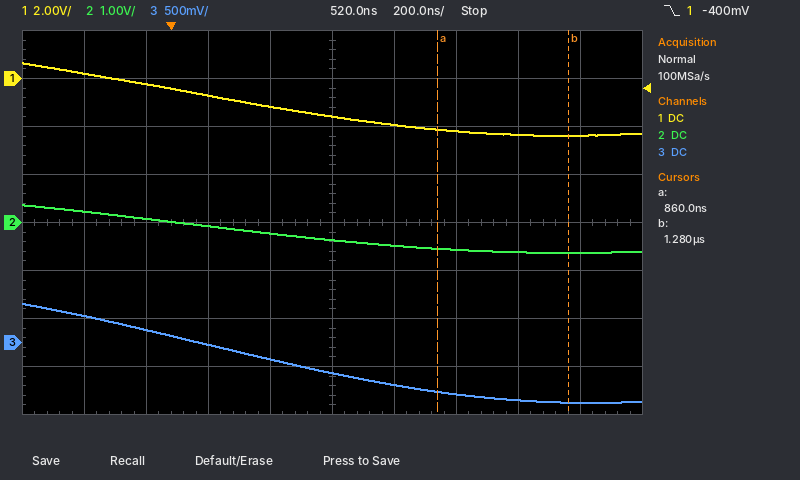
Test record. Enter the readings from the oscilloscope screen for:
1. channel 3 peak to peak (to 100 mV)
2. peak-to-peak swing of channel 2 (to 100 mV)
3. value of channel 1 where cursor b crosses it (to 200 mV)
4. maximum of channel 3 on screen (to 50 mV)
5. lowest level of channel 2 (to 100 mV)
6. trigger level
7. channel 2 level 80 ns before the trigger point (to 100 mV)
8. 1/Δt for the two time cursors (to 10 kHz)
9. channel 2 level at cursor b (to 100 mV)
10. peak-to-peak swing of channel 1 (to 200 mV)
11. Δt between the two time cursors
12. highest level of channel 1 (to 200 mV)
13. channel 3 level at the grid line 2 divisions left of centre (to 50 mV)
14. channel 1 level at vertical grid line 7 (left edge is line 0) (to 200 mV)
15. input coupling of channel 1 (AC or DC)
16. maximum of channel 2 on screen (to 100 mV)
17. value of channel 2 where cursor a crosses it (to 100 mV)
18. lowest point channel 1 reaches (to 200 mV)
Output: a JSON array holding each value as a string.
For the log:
["1.00 V", "1.0 V", "-2.4 V", "400 mV", "-600 mV", "-400 mV", "100 mV", "2.38 MHz", "-600 mV", "3.0 V", "420 ns", "600 mV", "0 mV", "-2.2 V", "DC", "400 mV", "-500 mV", "-2.4 V"]
